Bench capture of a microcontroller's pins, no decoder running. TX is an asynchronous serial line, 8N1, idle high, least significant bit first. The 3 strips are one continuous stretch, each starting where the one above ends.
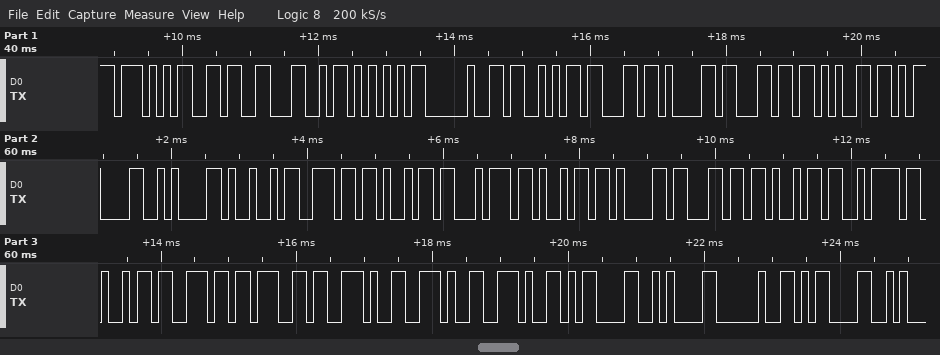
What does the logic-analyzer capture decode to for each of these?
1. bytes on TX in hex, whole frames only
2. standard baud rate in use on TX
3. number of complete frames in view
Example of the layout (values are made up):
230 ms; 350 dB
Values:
57 36 4C 55 20 53 63 61 6C 65 0D 0A 49 6E 69 74 69 61 6C 69 7A 69 6E 67 2E 2E 2E 0D 0A 20 0D; 9600 baud; 31
